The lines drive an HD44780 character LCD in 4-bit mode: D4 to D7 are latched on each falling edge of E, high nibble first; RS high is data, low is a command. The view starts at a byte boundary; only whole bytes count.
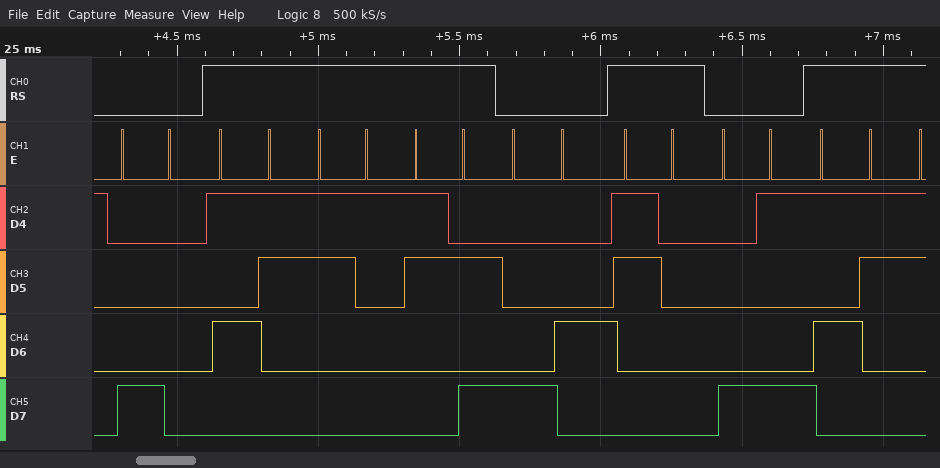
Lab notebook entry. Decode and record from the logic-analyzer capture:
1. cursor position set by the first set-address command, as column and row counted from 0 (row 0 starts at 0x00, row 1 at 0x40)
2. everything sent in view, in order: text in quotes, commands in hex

column 0, row 0
0x80 "S1:" 0x84 "0" 0x89 "S"
